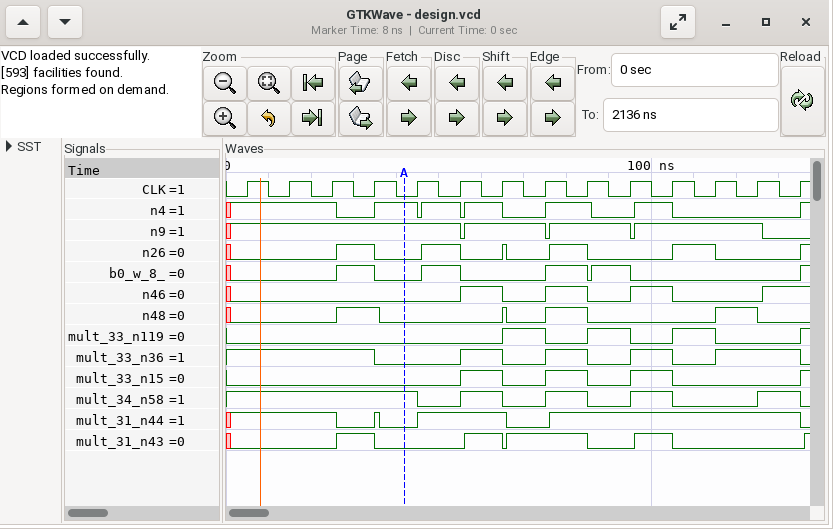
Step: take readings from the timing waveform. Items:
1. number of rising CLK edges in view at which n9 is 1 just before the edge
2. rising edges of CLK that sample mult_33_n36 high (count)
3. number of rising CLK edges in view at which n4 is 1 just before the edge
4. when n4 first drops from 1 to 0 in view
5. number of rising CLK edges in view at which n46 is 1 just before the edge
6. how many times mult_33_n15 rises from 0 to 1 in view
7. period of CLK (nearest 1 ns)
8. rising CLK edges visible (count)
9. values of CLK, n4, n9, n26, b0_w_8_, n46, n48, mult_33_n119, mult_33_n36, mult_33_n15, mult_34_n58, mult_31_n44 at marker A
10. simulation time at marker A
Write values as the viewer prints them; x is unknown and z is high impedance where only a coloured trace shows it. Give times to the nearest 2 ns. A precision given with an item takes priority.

13
9
8
26 ns
4
4
10 ns
14
CLK=0, n4=1, n9=1, n26=0, b0_w_8_=0, n46=0, n48=0, mult_33_n119=0, mult_33_n36=0, mult_33_n15=0, mult_34_n58=1, mult_31_n44=0
42 ns
